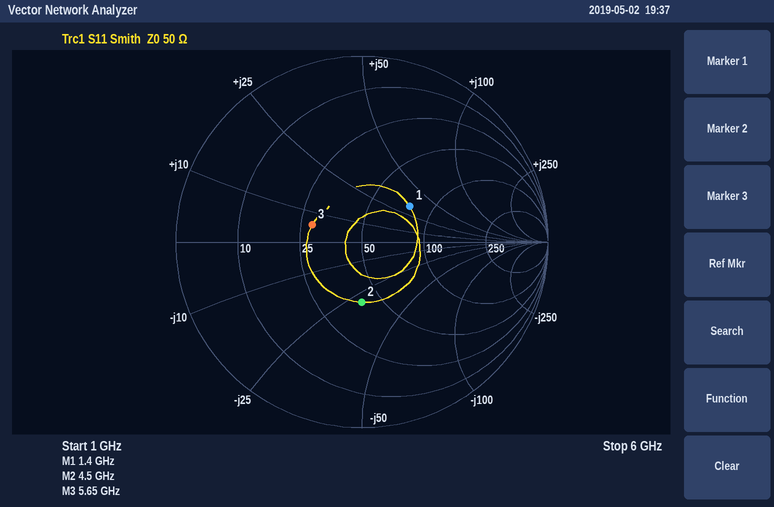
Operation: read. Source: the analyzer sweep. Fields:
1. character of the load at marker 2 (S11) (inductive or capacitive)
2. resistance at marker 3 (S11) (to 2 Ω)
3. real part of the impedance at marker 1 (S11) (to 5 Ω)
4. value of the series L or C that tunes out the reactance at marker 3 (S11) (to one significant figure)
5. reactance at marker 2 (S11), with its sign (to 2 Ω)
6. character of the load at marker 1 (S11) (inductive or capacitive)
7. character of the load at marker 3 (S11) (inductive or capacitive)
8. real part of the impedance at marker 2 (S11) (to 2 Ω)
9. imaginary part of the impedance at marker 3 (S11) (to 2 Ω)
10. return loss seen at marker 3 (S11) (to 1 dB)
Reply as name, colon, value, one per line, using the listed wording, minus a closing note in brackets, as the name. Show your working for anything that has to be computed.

character of the load at marker 2 (S11): capacitive
resistance at marker 3 (S11): 28 Ω
real part of the impedance at marker 1 (S11): 75 Ω
value of the series L or C that tunes out the reactance at marker 3 (S11): C = 1/(2π × 5.65 GHz × 6 Ω) ≈ 5 pF
reactance at marker 2 (S11), with its sign: -30 Ω
character of the load at marker 1 (S11): inductive
character of the load at marker 3 (S11): inductive
real part of the impedance at marker 2 (S11): 40 Ω
imaginary part of the impedance at marker 3 (S11): +6 Ω
return loss seen at marker 3 (S11): 11 dB
